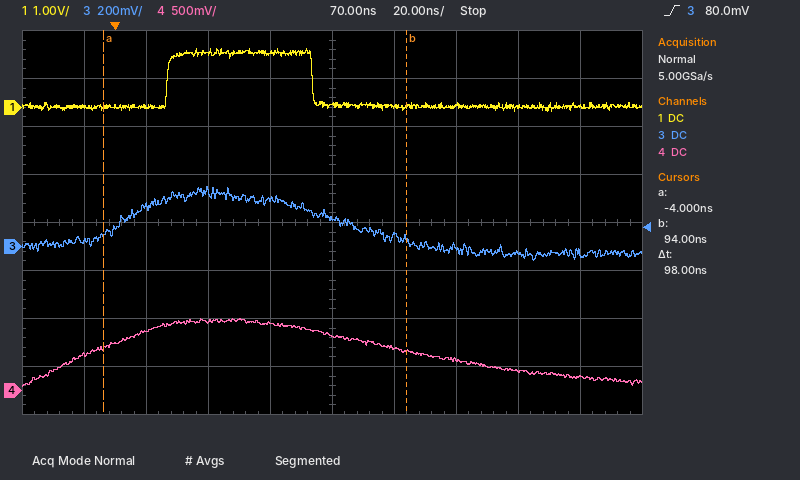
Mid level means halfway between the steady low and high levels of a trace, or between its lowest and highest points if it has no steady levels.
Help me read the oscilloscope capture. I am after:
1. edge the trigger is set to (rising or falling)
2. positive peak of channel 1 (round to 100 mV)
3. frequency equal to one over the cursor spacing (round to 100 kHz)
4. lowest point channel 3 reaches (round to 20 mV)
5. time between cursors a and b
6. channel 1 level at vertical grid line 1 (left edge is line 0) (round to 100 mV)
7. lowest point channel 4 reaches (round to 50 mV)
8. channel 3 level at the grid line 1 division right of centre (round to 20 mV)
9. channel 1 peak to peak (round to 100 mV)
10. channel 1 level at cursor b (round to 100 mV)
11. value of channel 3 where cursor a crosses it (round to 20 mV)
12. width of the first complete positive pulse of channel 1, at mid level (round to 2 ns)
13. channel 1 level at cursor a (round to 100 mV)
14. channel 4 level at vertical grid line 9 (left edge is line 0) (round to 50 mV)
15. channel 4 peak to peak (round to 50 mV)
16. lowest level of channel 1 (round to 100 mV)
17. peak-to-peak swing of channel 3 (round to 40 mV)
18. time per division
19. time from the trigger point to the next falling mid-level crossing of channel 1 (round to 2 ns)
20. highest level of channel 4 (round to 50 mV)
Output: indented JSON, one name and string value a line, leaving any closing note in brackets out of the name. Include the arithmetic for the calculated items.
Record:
{
  "edge the trigger is set to": "rising",
  "positive peak of channel 1": "1.2 V",
  "frequency equal to one over the cursor spacing": "1 / 98 ns ≈ 10.2 MHz",
  "lowest point channel 3 reaches": "-60 mV",
  "time between cursors a and b": "98 ns",
  "channel 1 level at vertical grid line 1 (left edge is line 0)": "0.0 V",
  "lowest point channel 4 reaches": "50 mV",
  "channel 3 level at the grid line 1 division right of centre": "40 mV",
  "channel 1 peak to peak": "1.2 V − (-100 mV) = 1.3 V",
  "channel 1 level at cursor b": "0.0 V",
  "value of channel 3 where cursor a crosses it": "60 mV",
  "width of the first complete positive pulse of channel 1, at mid level": "46 ns",
  "channel 1 level at cursor a": "0.0 V",
  "channel 4 level at vertical grid line 9 (left edge is line 0)": "150 mV",
  "channel 4 peak to peak": "750 mV − (50 mV) = 700 mV",
  "lowest level of channel 1": "-100 mV",
  "peak-to-peak swing of channel 3": "320 mV",
  "time per division": "20 ns",
  "time from the trigger point to the next falling mid-level crossing of channel 1": "64 ns",
  "highest level of channel 4": "750 mV"
}
